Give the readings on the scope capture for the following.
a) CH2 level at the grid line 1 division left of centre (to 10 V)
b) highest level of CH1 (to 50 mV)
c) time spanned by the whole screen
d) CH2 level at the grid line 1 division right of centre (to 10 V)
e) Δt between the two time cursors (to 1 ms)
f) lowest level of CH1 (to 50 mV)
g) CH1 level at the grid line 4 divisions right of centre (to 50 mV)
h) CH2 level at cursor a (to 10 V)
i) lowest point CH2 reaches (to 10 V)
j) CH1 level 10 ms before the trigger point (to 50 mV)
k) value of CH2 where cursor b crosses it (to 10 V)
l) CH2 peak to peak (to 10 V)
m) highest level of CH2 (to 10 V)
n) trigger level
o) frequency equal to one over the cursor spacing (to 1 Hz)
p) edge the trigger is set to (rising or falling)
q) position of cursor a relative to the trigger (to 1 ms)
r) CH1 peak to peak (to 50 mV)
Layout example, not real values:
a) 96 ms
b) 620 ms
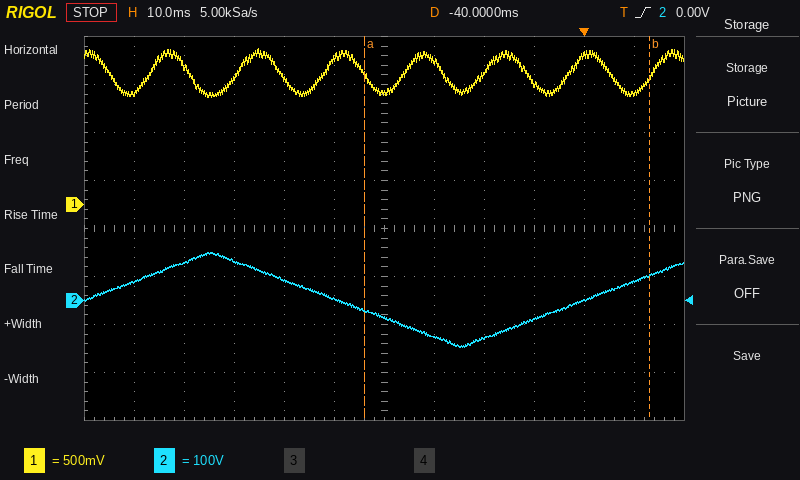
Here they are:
a) 0 V
b) 1.60 V
c) 120 ms
d) -80 V
e) 57 ms
f) 1.10 V
g) 1.55 V
h) -20 V
i) -100 V
j) 1.25 V
k) 50 V
l) 200 V
m) 100 V
n) 0.00 V
o) 18 Hz
p) rising
q) -44 ms
r) 500 mV
